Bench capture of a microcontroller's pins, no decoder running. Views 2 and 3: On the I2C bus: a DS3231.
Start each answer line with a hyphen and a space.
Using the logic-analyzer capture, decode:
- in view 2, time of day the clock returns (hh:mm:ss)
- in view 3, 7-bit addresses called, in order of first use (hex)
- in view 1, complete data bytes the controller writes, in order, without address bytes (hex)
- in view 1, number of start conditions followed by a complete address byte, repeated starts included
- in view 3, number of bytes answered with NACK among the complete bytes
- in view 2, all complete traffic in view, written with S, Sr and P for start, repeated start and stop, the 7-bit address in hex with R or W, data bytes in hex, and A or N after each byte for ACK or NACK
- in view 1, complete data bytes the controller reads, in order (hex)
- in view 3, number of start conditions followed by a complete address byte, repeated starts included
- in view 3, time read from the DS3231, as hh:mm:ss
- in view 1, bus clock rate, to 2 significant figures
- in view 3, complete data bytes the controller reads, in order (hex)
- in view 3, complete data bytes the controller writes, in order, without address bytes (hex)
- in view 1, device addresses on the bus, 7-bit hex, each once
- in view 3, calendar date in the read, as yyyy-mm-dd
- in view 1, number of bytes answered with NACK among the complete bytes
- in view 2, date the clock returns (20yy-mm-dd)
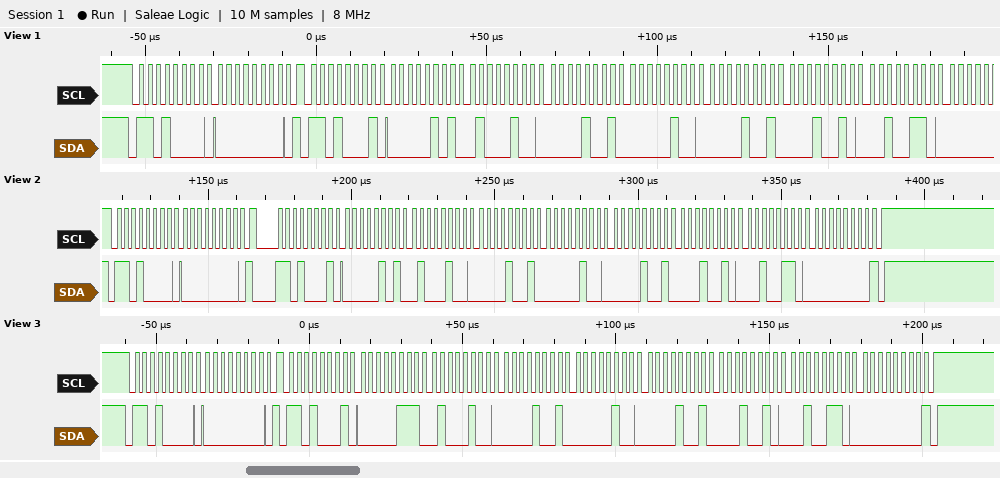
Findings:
- 09:44:05
- 0x68
- 00
- 2
- 1
- S 68W A 00 A Sr 68R A 05 A 44 A 09 A 04 A 09 A 12 A 26 A 00 N P
- 05 44 09 04 09 12 26
- 2
- 09:44:07
- 400 kHz
- 07 44 09 04 09 12 26 00
- 00
- 0x68
- 2026-12-09
- 0
- 2026-12-09
